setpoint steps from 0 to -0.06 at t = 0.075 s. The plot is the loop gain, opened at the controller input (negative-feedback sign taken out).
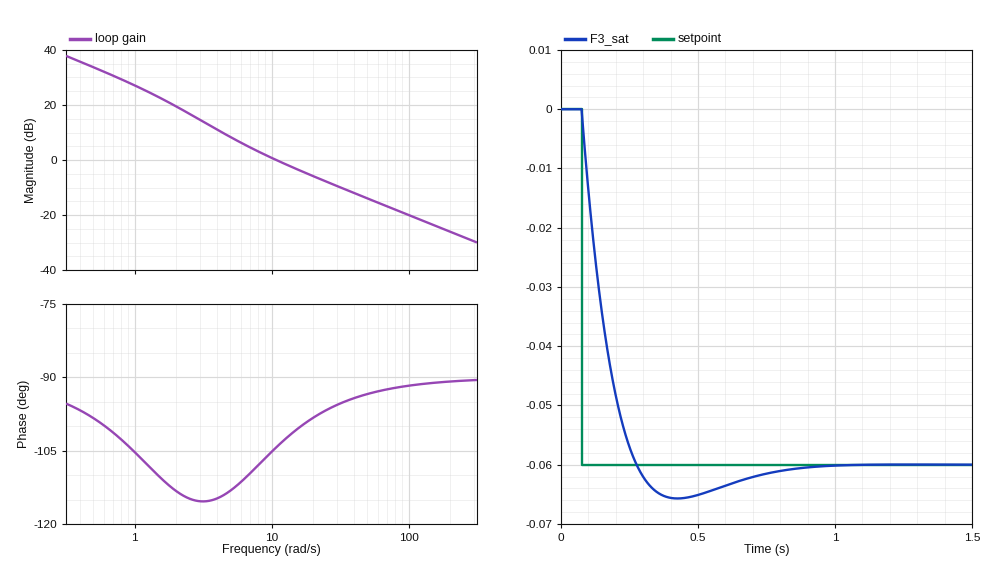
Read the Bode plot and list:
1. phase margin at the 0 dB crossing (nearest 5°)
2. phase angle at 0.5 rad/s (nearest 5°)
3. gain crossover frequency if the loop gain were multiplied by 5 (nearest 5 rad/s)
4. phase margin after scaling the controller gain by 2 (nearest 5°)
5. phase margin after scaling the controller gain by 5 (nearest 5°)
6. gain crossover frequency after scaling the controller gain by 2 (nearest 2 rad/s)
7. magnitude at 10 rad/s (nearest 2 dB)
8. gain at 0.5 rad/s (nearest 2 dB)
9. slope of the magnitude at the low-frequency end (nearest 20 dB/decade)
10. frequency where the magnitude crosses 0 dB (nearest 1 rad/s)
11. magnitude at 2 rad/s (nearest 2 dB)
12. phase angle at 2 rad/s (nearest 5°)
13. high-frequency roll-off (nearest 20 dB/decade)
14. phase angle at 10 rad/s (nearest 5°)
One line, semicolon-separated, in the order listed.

75°; -100°; 50 rad/s; 80°; 85°; 20 rad/s; 0 dB; 34 dB; -20 dB/decade; 11 rad/s; 20 dB; -115°; -20 dB/decade; -105°
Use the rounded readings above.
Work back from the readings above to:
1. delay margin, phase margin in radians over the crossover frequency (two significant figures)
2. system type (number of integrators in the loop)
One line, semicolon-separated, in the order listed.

0.12 s; 1
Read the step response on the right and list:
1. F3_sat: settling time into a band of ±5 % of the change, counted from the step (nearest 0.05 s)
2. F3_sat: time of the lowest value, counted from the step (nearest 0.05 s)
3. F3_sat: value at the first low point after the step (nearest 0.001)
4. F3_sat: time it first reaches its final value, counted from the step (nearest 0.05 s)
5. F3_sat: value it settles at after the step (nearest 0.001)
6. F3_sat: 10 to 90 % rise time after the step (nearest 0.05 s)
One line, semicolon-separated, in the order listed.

0.55 s; 0.35 s; -0.066; 0.20 s; -0.060; 0.15 s
